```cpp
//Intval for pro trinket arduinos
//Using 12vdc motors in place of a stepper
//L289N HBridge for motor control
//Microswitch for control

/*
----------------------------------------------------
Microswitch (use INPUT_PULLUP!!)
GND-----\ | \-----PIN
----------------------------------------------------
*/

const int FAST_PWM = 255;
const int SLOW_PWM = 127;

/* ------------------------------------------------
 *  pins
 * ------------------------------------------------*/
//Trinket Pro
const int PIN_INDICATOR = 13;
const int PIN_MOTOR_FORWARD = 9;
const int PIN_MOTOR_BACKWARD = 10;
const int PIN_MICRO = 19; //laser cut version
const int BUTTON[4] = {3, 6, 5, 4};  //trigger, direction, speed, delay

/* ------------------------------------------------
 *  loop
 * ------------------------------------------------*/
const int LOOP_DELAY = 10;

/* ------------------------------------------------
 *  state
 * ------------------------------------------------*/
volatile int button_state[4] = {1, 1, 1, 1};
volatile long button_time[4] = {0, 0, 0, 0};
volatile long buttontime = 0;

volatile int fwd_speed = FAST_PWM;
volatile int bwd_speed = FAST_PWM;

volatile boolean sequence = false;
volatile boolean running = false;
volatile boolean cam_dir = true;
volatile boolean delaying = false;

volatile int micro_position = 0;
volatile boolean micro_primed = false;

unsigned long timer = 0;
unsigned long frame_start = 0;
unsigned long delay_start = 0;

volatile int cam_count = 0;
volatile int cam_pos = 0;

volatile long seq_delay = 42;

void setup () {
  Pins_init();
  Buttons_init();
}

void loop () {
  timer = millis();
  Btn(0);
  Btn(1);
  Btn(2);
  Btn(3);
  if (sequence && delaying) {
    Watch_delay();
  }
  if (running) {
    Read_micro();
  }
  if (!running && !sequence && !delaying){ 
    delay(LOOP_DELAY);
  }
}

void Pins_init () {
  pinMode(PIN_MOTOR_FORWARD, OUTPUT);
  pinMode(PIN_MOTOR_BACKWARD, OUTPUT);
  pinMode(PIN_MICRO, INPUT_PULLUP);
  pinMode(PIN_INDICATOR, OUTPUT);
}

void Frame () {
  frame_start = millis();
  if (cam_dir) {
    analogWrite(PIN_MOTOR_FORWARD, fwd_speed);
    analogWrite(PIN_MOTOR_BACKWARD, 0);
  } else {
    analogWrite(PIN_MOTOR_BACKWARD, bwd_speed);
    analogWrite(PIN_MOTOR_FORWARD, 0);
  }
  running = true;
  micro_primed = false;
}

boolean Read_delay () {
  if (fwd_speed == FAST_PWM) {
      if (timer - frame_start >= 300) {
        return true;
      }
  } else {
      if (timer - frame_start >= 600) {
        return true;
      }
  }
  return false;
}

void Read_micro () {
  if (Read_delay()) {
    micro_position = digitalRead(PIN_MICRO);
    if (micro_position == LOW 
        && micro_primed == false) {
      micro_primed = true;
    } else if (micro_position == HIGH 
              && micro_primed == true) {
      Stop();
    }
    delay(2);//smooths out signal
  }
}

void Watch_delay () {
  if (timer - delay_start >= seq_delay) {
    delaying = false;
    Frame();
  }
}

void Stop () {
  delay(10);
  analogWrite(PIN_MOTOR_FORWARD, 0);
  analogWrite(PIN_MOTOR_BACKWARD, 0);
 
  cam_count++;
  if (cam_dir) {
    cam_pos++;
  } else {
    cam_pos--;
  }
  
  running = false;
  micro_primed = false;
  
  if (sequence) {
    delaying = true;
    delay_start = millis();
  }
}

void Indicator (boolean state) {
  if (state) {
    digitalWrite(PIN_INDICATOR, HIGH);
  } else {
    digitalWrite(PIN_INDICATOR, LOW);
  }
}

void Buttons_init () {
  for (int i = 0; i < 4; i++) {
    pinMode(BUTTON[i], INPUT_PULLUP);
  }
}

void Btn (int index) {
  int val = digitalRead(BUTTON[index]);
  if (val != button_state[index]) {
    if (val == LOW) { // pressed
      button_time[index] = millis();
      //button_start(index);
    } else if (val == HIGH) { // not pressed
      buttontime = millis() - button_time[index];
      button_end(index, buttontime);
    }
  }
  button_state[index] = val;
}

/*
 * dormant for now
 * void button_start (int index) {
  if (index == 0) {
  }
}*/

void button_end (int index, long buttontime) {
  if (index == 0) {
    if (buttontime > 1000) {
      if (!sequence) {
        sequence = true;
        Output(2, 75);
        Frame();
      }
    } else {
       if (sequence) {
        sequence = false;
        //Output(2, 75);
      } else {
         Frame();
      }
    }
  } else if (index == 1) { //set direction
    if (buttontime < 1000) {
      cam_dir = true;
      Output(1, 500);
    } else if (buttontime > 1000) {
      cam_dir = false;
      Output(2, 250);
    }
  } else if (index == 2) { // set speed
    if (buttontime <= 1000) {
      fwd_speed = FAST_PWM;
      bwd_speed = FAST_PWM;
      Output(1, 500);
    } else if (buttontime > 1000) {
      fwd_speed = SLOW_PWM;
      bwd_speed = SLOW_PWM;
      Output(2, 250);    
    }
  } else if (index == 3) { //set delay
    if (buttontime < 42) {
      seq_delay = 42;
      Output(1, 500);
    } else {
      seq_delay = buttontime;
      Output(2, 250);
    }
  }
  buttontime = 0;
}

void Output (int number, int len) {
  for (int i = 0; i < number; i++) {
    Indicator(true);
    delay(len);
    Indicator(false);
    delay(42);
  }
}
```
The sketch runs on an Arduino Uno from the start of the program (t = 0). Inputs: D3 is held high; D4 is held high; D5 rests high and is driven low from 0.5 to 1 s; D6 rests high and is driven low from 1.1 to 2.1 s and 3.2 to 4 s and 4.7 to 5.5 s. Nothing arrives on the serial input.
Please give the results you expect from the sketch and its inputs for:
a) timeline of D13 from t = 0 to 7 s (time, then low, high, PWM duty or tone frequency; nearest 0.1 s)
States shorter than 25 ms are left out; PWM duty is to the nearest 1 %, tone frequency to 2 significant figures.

0 s low; 1 s high; 1.5 s low; 2.1 s high; 2.6 s low; 4 s high; 4.5 s low; 5.5 s high; 6 s low
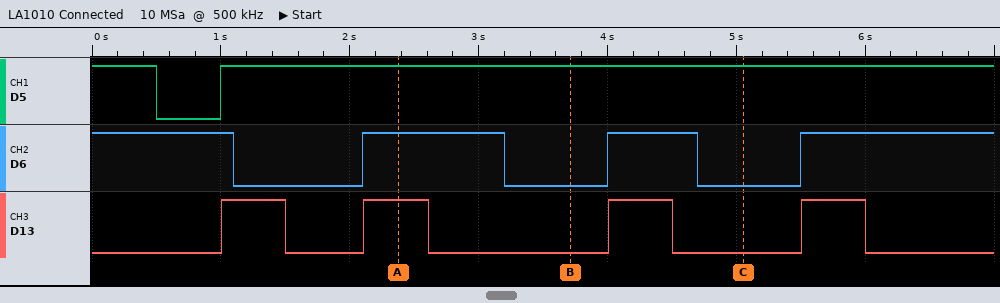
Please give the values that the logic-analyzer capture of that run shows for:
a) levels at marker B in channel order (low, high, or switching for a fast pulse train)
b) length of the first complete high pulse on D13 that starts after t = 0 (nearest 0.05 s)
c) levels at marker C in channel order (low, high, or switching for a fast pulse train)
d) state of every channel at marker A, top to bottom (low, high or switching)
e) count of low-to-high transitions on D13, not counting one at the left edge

D5 high, D6 low, D13 low
0.50 s
D5 high, D6 low, D13 low
D5 high, D6 high, D13 high
4
